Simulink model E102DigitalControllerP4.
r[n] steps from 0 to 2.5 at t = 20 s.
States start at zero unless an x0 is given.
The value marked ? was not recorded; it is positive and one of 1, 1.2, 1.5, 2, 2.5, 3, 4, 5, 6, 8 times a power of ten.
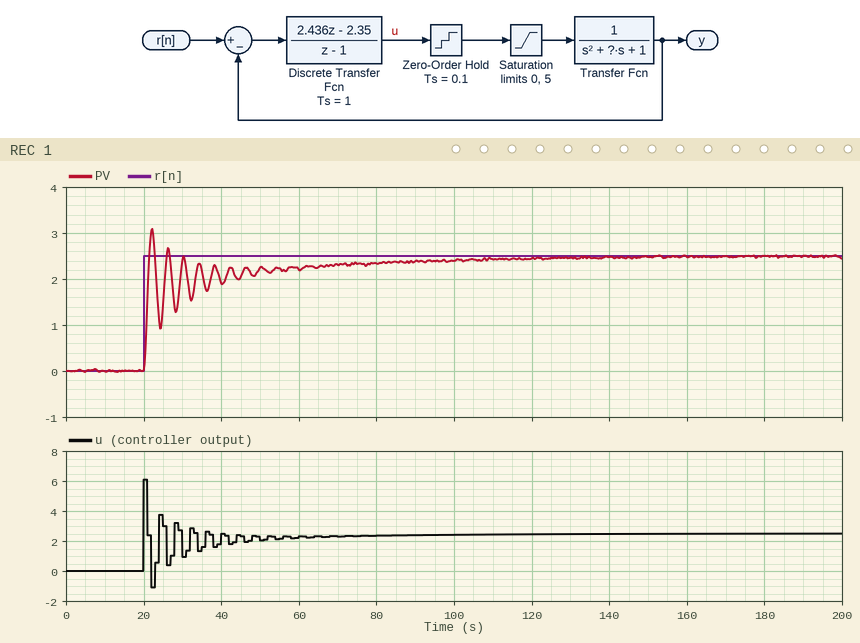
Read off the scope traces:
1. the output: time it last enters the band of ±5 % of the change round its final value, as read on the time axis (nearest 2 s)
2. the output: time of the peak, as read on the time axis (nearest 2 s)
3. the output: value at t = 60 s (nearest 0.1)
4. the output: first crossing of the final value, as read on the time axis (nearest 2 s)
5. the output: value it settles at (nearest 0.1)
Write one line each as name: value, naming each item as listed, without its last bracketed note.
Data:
the output: time it last enters the band of ±5 % of the change round its final value, as read on the time axis: 88 s
the output: time of the peak, as read on the time axis: 22 s
the output: value at t = 60 s: 2.2
the output: first crossing of the final value, as read on the time axis: 22 s
the output: value it settles at: 2.5
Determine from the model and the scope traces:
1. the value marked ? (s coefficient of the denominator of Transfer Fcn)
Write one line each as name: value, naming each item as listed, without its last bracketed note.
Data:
the value marked ?: 1.2
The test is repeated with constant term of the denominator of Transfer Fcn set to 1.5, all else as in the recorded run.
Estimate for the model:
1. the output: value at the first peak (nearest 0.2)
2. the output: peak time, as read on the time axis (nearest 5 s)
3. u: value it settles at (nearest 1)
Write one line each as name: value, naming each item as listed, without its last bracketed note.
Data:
the output: value at the first peak: 2.6
the output: peak time, as read on the time axis: 20 s
u: value it settles at: 4
